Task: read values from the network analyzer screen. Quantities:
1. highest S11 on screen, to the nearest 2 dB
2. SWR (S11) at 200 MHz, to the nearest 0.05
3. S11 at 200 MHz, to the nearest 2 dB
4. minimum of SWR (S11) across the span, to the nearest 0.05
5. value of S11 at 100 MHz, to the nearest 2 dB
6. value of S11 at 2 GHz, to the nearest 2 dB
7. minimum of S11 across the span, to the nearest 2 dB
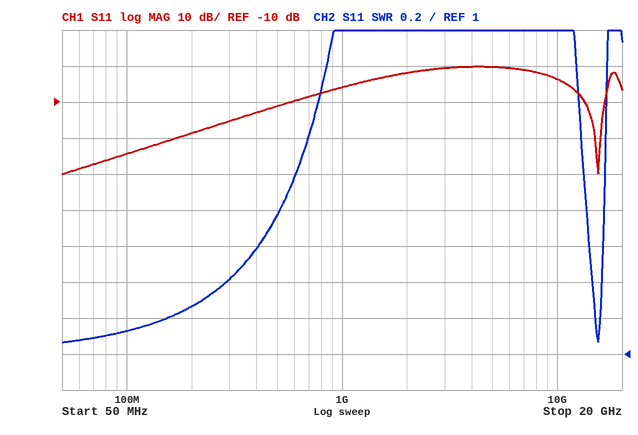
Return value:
0 dB
1.25
-18 dB
1.05
-24 dB
-2 dB
-30 dB
